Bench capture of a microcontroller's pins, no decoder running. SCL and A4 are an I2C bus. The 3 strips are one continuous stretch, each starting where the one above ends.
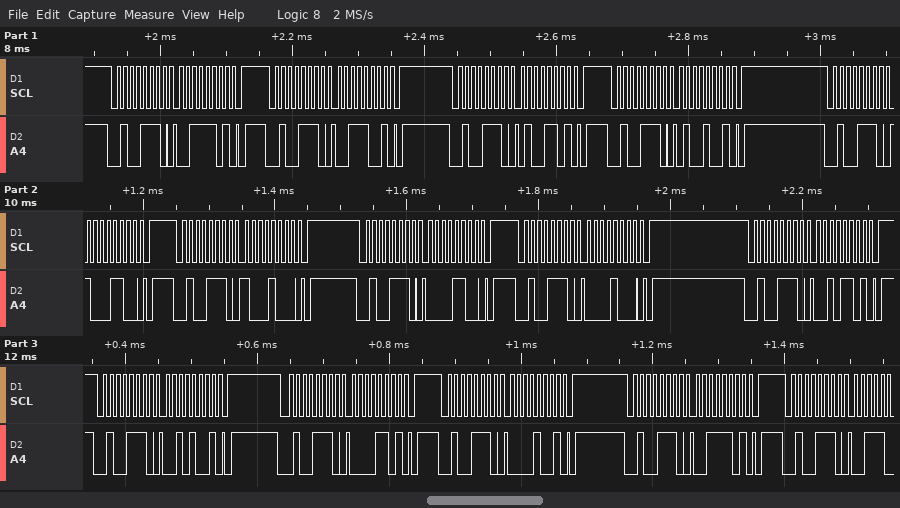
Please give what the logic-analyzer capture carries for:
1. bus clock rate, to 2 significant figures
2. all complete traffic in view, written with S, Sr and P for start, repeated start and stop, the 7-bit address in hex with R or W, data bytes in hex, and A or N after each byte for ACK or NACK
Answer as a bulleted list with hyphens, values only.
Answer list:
- 100 kHz
- S 27W A 3D A P S 27W A 39 A P S 27W A 4D A P S 27W A 49 A P S 27W A 8C A P S 27W A 88 A P S 27W A 0C A P S 27W A 08 A P S 27W A 2D A P S 27W A 29 A P S 27W A 0D A P S 27W A 09 A P S 27W A 3D A P S 27W A
